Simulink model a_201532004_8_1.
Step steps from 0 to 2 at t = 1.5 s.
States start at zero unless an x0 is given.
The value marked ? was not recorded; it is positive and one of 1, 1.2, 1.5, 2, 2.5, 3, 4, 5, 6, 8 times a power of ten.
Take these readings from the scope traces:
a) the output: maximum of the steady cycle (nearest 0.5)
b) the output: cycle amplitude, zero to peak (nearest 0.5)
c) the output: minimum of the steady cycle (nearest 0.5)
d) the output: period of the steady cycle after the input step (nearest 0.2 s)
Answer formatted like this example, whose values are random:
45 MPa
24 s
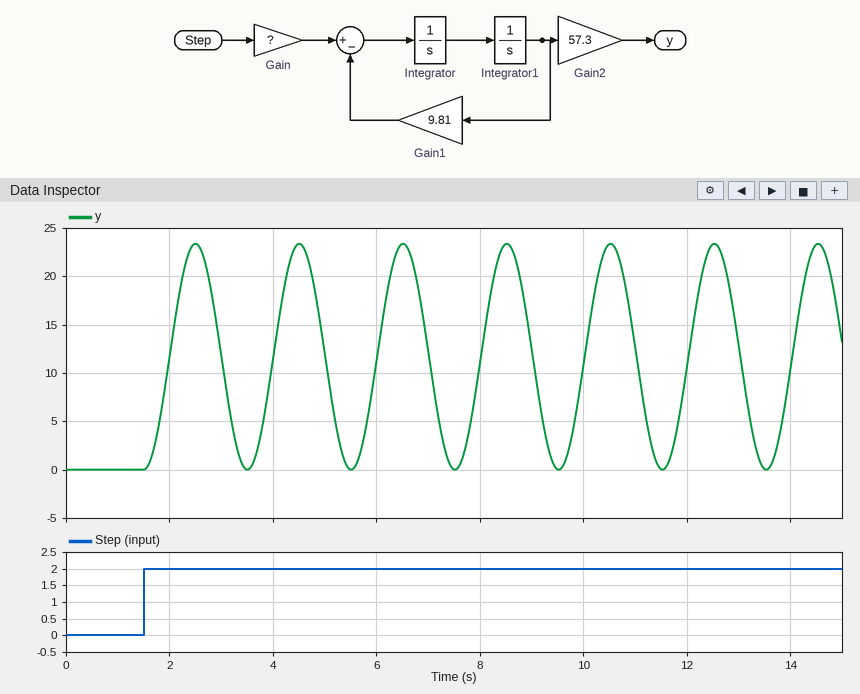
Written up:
23.5
11.5
0.0
2.0 s
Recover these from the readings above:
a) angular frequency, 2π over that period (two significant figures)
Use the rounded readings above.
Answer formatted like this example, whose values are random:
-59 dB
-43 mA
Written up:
3.1 rad/s
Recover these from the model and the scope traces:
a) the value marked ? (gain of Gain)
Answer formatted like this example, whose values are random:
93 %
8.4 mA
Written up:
1
